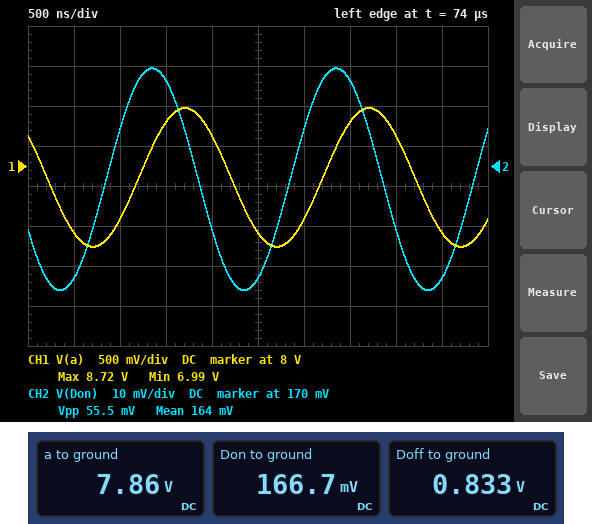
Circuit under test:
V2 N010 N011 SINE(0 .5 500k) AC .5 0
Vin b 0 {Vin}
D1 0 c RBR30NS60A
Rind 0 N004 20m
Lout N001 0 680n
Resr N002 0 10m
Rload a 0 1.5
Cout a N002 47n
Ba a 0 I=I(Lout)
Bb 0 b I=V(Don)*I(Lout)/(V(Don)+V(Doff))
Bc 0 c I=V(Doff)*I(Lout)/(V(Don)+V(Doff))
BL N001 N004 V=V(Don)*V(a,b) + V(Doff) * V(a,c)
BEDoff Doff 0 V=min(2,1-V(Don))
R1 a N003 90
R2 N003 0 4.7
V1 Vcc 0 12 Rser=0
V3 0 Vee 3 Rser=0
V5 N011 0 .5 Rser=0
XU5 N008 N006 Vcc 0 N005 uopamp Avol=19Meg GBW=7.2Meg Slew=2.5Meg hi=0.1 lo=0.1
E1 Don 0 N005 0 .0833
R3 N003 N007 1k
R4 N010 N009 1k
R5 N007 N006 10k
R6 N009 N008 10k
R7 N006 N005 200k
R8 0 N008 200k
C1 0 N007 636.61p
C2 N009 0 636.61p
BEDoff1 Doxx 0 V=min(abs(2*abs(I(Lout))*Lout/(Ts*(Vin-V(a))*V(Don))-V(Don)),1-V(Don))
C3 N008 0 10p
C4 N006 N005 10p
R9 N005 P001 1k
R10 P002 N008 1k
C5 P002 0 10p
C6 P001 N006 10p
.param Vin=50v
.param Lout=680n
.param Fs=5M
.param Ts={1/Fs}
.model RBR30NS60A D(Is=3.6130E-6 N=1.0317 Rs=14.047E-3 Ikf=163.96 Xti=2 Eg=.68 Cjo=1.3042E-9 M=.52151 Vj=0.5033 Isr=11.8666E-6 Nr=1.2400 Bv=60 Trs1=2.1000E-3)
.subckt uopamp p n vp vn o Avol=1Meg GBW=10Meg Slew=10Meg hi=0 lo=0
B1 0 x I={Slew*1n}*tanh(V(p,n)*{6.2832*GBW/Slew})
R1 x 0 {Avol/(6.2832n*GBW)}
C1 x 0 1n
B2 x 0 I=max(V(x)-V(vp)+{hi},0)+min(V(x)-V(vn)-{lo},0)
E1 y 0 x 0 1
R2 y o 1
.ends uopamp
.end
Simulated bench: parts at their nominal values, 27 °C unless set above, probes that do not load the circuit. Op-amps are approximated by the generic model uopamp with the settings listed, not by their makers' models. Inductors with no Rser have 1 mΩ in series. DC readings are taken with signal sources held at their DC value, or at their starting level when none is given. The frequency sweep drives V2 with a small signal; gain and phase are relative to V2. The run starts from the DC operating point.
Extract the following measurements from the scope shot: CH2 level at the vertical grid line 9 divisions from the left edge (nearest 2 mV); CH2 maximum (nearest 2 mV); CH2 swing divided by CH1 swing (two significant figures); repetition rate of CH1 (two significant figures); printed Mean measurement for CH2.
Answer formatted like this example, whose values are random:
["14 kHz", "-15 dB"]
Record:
["142 mV", "194 mV", "0.032", "500 kHz", "164 mV"]
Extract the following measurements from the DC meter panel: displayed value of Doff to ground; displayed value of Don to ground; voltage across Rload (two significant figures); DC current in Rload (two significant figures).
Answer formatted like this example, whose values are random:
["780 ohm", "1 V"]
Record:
["0.833 V", "166.7 mV", "7.9 V", "5.2 A"]
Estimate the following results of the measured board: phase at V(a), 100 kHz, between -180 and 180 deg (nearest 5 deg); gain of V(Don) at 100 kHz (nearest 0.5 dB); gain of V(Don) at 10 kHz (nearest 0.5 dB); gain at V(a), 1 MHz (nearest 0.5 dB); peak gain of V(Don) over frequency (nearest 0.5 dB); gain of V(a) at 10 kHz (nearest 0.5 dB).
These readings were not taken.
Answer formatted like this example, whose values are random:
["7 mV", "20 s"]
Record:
["-50 deg", "-8.5 dB", "-10.0 dB", "-12.0 dB", "-8.0 dB", "24.0 dB"]
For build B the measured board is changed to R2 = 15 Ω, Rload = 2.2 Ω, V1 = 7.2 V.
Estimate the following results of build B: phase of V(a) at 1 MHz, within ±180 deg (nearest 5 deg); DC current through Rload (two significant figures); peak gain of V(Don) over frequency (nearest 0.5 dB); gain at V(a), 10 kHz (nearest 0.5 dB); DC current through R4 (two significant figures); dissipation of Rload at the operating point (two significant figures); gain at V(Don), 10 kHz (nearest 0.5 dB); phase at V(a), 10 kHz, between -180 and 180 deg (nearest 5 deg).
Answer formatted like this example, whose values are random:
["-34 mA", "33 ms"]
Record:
["90 deg", "1.4 A", "-7.5 dB", "16.0 dB", "2.4 µA", "4.6 W", "-17.5 dB", "0 deg"]
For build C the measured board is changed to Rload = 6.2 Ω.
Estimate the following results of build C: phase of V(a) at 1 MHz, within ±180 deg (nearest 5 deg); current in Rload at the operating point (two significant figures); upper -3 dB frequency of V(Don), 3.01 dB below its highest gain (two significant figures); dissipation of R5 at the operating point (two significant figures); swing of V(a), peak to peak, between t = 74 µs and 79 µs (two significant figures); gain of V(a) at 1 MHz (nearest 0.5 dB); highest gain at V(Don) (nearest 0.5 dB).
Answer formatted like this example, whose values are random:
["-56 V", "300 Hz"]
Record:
["80 deg", "1.3 A", "240 kHz", "560 nW", "4.0 V", "-1.0 dB", "-10.0 dB"]
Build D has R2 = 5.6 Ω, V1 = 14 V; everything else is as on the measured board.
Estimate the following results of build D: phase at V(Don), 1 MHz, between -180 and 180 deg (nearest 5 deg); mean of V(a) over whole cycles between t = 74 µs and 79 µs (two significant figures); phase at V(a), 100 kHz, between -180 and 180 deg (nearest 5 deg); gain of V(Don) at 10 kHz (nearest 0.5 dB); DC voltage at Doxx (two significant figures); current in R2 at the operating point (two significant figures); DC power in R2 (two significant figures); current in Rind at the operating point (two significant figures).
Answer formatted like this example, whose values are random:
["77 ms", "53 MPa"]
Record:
["-170 deg", "6.9 V", "-40 deg", "-11.0 dB", "150 mV", "72 mA", "29 mW", "4.7 A"]
